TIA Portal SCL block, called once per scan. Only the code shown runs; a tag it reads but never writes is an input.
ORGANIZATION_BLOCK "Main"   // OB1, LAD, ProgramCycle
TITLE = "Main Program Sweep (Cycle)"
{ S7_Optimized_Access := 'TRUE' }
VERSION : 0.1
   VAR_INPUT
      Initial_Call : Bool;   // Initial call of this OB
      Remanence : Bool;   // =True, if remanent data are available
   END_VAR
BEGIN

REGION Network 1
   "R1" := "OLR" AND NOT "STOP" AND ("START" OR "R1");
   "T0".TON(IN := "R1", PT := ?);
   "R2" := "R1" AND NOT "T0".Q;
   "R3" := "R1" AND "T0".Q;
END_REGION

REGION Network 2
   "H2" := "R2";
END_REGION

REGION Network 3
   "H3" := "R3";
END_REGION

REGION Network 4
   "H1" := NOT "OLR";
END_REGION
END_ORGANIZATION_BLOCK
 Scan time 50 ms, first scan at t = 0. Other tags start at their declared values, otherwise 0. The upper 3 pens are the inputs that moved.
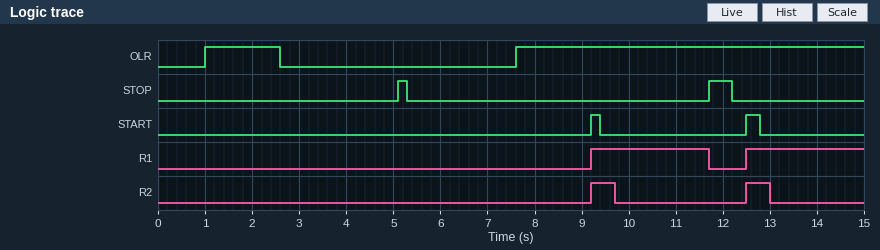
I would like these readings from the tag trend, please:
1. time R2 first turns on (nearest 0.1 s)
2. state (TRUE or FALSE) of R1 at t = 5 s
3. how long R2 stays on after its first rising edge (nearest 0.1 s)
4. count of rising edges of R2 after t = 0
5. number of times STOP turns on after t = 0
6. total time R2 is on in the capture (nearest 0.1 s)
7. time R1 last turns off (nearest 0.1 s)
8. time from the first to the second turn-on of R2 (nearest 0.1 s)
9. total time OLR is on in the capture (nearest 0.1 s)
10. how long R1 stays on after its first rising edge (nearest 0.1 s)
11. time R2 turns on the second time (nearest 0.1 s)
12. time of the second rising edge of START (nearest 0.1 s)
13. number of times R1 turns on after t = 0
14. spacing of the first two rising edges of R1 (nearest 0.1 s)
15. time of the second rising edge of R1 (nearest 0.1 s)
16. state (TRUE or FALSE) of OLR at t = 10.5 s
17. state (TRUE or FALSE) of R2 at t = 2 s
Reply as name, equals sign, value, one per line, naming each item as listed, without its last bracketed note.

time R2 first turns on = 9.2 s
state (TRUE or FALSE) of R1 at t = 5 s = FALSE
how long R2 stays on after its first rising edge = 0.5 s
count of rising edges of R2 after t = 0 = 2
number of times STOP turns on after t = 0 = 2
total time R2 is on in the capture = 1.0 s
time R1 last turns off = 11.7 s
time from the first to the second turn-on of R2 = 3.3 s
total time OLR is on in the capture = 9.0 s
how long R1 stays on after its first rising edge = 2.5 s
time R2 turns on the second time = 12.5 s
time of the second rising edge of START = 12.5 s
number of times R1 turns on after t = 0 = 2
spacing of the first two rising edges of R1 = 3.3 s
time of the second rising edge of R1 = 12.5 s
state (TRUE or FALSE) of OLR at t = 10.5 s = TRUE
state (TRUE or FALSE) of R2 at t = 2 s = FALSE
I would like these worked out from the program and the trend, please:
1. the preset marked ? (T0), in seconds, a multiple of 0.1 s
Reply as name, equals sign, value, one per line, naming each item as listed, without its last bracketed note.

the preset marked ? (T0), in seconds, a multiple of 0.1 s = 0.5 s
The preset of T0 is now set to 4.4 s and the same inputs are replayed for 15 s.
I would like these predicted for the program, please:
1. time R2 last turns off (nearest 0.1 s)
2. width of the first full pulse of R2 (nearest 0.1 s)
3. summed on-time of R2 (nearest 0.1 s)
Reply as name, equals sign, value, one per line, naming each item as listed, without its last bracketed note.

time R2 last turns off = 11.7 s
width of the first full pulse of R2 = 2.5 s
summed on-time of R2 = 5.0 s
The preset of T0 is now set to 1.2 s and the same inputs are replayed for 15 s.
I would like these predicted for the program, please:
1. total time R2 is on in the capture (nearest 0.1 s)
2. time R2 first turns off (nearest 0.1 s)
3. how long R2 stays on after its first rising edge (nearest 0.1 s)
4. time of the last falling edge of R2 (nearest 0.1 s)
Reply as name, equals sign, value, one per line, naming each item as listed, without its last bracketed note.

total time R2 is on in the capture = 2.4 s
time R2 first turns off = 10.4 s
how long R2 stays on after its first rising edge = 1.2 s
time of the last falling edge of R2 = 13.7 s
